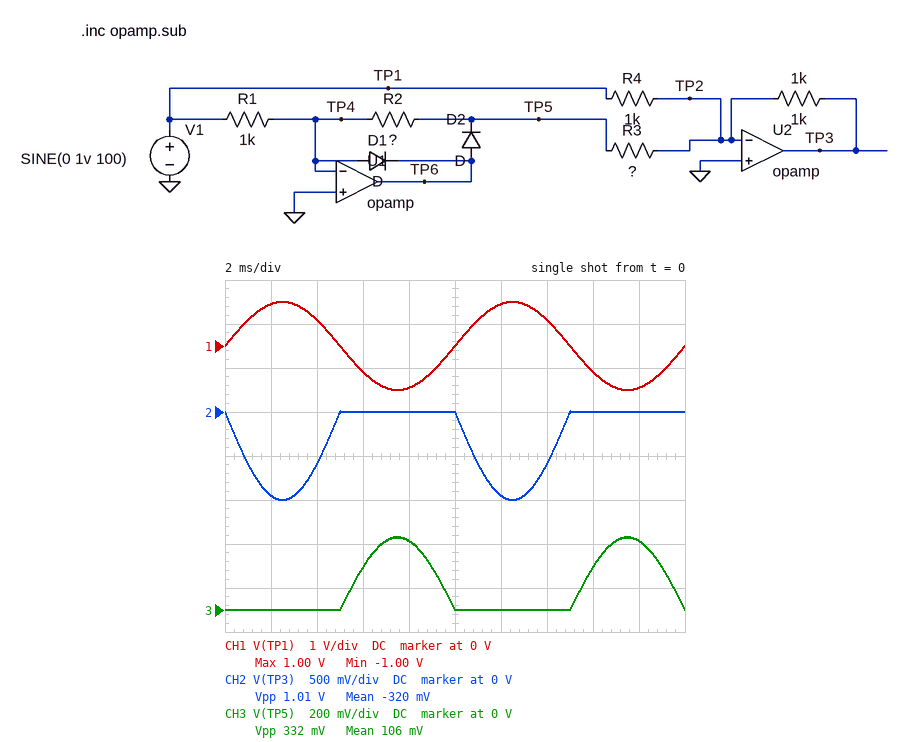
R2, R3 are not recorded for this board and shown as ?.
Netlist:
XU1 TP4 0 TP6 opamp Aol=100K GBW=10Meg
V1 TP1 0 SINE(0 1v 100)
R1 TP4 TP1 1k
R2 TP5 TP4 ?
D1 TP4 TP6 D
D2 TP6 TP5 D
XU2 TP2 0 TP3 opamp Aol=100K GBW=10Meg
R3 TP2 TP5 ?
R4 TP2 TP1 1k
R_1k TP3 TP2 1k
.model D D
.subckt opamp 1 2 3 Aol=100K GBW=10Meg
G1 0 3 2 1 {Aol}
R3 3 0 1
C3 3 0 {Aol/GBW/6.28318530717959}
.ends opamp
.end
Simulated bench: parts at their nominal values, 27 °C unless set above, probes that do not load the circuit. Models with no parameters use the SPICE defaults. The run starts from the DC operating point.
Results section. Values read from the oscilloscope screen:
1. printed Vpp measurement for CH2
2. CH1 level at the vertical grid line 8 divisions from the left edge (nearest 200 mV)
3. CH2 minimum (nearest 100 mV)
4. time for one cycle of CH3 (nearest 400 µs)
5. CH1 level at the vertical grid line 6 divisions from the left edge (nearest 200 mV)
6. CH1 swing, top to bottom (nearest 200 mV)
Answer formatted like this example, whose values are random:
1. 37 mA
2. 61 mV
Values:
1. 1.01 V
2. -600 mV
3. -1.0 V
4. 10.0 ms
5. 1.0 V
6. 2.0 V
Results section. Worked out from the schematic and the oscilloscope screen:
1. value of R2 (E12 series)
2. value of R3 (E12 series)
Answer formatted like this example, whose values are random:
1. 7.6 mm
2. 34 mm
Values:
1. 330 Ω
2. 330 Ω
